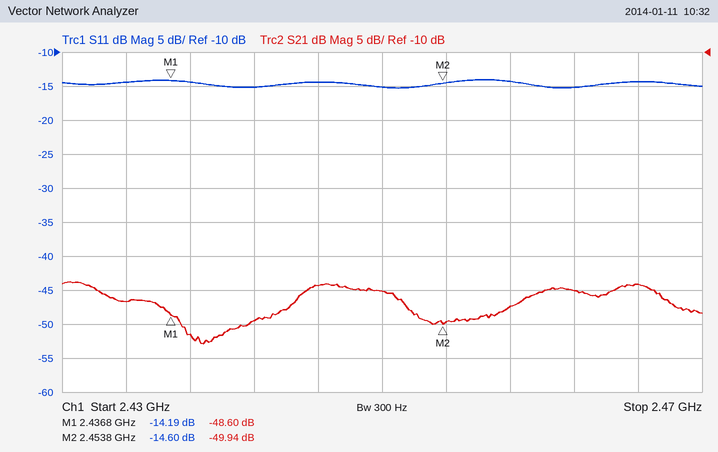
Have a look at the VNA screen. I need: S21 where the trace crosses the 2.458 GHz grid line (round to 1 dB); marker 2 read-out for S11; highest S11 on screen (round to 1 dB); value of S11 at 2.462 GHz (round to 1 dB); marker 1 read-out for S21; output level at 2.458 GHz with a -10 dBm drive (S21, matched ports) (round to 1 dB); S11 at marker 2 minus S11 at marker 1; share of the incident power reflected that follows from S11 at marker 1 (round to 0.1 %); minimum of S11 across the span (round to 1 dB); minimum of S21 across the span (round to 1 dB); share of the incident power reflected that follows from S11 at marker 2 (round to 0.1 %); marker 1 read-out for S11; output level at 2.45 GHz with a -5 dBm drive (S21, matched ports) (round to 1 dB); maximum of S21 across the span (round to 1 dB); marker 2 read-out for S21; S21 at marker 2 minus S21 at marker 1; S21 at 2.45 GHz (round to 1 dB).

-47 dB
-14.60 dB
-14 dB
-15 dB
-48.60 dB
-57 dBm
-0.41 dB
3.8 %
-15 dB
-53 dB
3.5 %
-14.19 dB
-50 dBm
-44 dB
-49.94 dB
-1.34 dB
-45 dB
